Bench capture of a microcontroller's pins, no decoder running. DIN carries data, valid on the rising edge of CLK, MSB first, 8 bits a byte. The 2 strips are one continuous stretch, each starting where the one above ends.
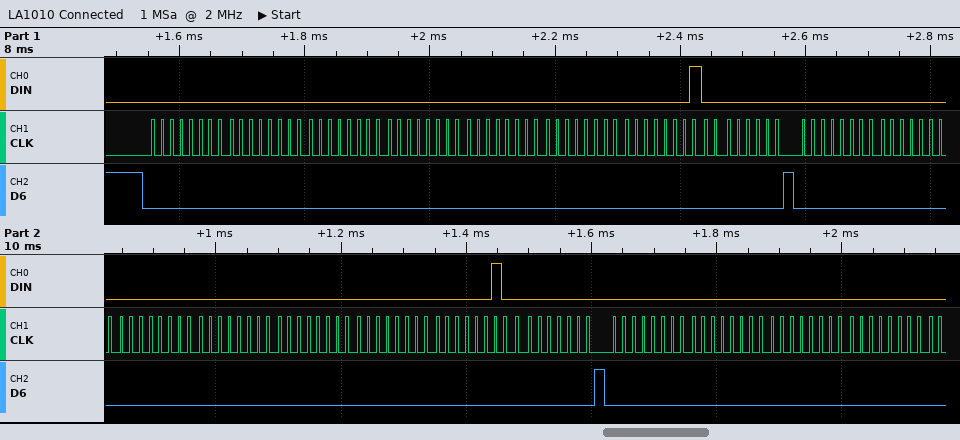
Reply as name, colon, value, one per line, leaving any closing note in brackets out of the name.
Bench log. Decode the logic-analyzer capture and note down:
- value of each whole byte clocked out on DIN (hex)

value of each whole byte clocked out on DIN: 00 00 00 00 00 00 01 00 00 00 00 00 00 00 02 00 00 00 00 00
